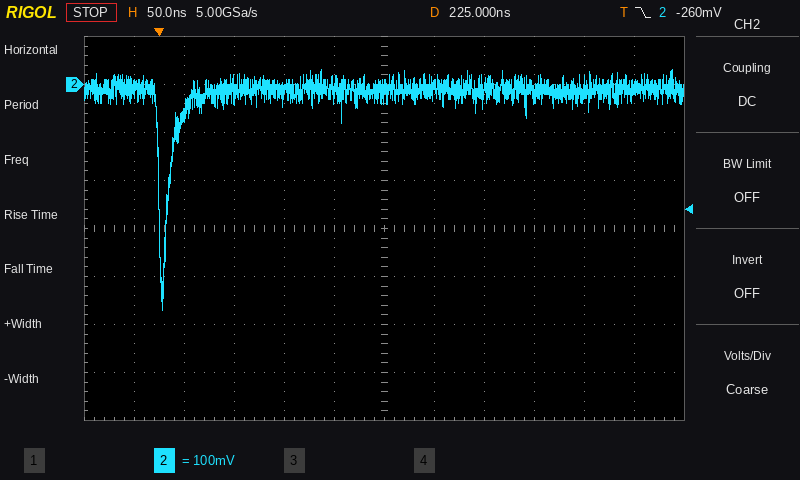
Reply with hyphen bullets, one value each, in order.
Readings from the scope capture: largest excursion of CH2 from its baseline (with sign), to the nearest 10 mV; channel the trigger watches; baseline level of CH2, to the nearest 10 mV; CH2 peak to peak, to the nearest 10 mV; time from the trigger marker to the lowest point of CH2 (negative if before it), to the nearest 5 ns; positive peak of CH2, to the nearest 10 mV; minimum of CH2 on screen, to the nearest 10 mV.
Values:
- -460 mV
- CH2
- -10 mV
- 500 mV
- +5 ns
- 30 mV
- -470 mV
